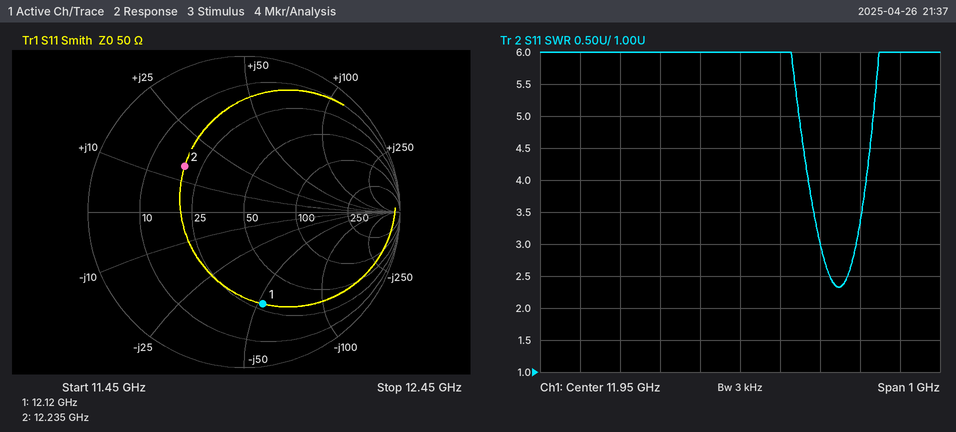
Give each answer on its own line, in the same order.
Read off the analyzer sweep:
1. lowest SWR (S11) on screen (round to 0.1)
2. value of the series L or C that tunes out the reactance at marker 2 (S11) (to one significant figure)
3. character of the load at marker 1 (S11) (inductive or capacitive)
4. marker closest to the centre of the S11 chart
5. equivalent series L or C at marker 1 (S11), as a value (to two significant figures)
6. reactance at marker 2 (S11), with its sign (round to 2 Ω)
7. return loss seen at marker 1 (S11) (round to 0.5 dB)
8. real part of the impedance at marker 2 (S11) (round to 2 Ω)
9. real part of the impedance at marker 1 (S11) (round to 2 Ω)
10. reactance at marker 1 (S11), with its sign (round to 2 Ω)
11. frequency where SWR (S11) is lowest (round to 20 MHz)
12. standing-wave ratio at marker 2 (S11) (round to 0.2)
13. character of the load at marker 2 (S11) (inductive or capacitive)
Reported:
2.3
900 fF
capacitive
marker 2
250 fF
+14 Ω
4.5 dB
20 Ω
28 Ω
-52 Ω
12.20 GHz
2.8
inductive
